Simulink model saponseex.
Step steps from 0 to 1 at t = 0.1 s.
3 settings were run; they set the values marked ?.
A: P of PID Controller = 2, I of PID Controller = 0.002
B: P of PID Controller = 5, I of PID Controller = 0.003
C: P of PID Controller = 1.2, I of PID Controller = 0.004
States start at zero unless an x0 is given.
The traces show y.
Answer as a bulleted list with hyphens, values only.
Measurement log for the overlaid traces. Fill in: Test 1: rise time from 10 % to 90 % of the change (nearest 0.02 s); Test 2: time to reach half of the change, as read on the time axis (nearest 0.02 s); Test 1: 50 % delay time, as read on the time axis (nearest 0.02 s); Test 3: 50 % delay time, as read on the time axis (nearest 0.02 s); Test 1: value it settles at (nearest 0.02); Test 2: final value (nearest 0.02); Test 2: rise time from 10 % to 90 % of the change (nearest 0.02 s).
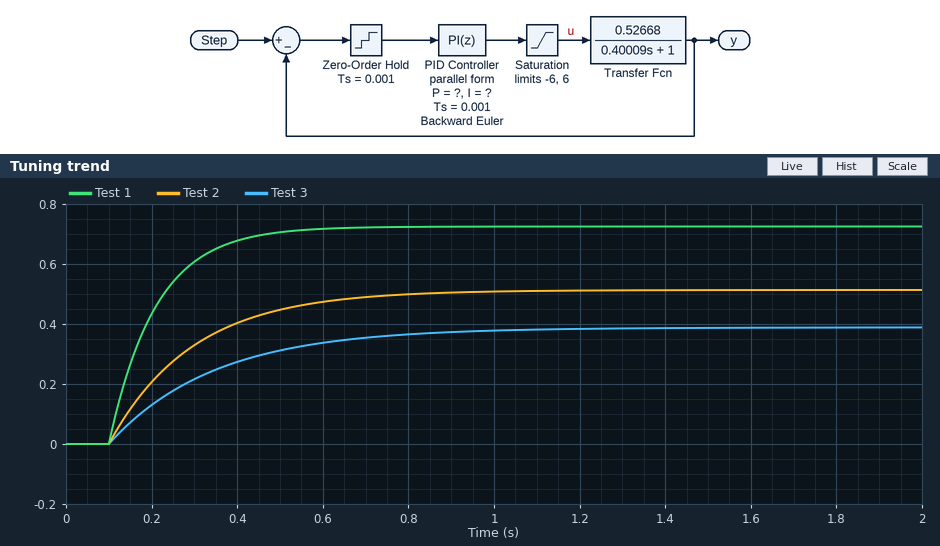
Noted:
- 0.24 s
- 0.24 s
- 0.18 s
- 0.28 s
- 0.72
- 0.52
- 0.44 s
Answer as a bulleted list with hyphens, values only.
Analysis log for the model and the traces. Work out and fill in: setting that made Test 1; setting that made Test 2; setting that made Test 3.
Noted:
- B
- A
- C
